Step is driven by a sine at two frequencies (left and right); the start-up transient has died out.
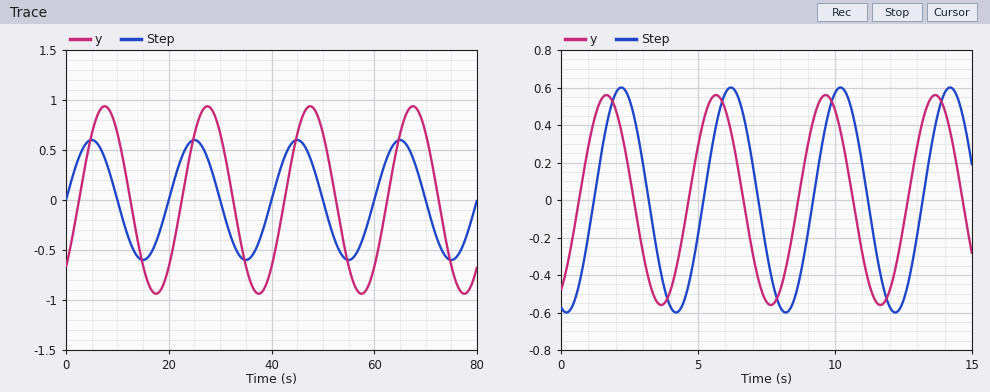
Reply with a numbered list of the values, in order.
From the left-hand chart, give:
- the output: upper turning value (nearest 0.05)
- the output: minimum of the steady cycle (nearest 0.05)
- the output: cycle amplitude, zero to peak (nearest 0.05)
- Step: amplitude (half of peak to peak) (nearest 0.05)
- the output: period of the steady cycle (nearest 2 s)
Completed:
1. 0.95
2. -0.95
3. 0.95
4. 0.60
5. 20 s
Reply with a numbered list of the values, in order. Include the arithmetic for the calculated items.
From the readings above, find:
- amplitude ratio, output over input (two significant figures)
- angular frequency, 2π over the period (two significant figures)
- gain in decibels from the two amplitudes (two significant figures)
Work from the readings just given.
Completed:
1. 0.95 / 0.6 = 1.6
2. 2π / 20 = 0.31 rad/s
3. 20 log10(0.95 / 0.6) = 4.0 dB
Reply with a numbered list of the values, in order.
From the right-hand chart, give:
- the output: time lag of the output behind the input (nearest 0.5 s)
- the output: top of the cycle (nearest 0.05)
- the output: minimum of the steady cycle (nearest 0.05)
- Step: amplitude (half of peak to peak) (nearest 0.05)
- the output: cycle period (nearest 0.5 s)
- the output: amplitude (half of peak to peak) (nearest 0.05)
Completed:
1. 3.5 s
2. 0.55
3. -0.55
4. 0.60
5. 4.0 s
6. 0.55
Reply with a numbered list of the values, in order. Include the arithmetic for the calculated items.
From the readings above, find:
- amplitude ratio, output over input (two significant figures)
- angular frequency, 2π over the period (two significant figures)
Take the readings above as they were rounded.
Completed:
1. 0.55 / 0.6 = 0.92
2. 2π / 4 = 1.6 rad/s
